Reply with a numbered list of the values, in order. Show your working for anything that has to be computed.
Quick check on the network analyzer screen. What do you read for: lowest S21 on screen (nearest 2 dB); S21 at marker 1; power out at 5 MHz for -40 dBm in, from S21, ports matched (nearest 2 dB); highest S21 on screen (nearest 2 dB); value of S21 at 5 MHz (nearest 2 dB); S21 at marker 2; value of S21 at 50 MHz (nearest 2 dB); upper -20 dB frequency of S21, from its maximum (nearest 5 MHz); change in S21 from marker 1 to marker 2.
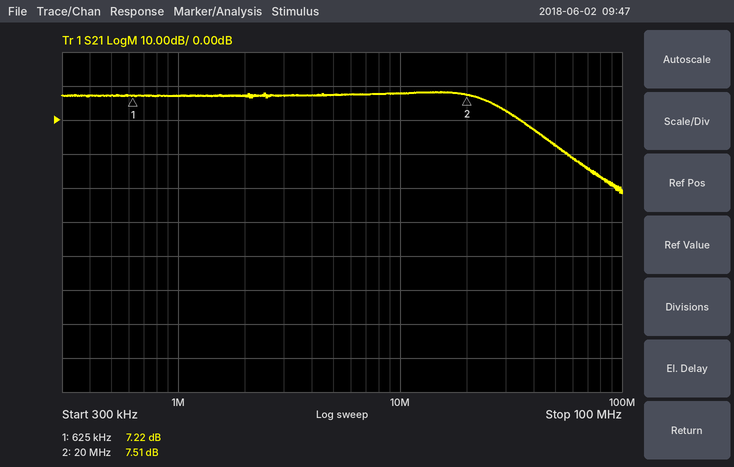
1. -22 dB
2. 7.22 dB
3. -40 dBm + (8 dB) = -32 dBm
4. 8 dB
5. 8 dB
6. 7.51 dB
7. -8 dB
8. 60 MHz
9. 7.51 − (7.22) = 0.29 dB
